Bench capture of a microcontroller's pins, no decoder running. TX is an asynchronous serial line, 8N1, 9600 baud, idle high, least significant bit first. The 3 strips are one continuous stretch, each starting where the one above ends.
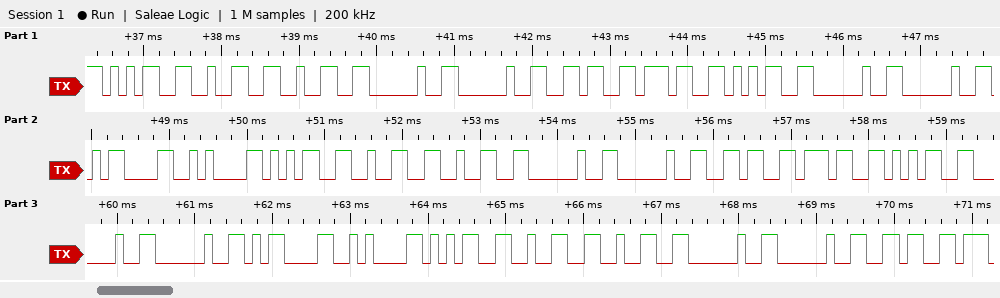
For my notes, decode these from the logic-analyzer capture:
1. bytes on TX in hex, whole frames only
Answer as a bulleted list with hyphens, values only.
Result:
- 35 32 32 20 20 36 37 35 20 20 0D 0A 35 32 32 20 20 36 37 35 20 20 0D 0A 35 32 32 20 20 36
